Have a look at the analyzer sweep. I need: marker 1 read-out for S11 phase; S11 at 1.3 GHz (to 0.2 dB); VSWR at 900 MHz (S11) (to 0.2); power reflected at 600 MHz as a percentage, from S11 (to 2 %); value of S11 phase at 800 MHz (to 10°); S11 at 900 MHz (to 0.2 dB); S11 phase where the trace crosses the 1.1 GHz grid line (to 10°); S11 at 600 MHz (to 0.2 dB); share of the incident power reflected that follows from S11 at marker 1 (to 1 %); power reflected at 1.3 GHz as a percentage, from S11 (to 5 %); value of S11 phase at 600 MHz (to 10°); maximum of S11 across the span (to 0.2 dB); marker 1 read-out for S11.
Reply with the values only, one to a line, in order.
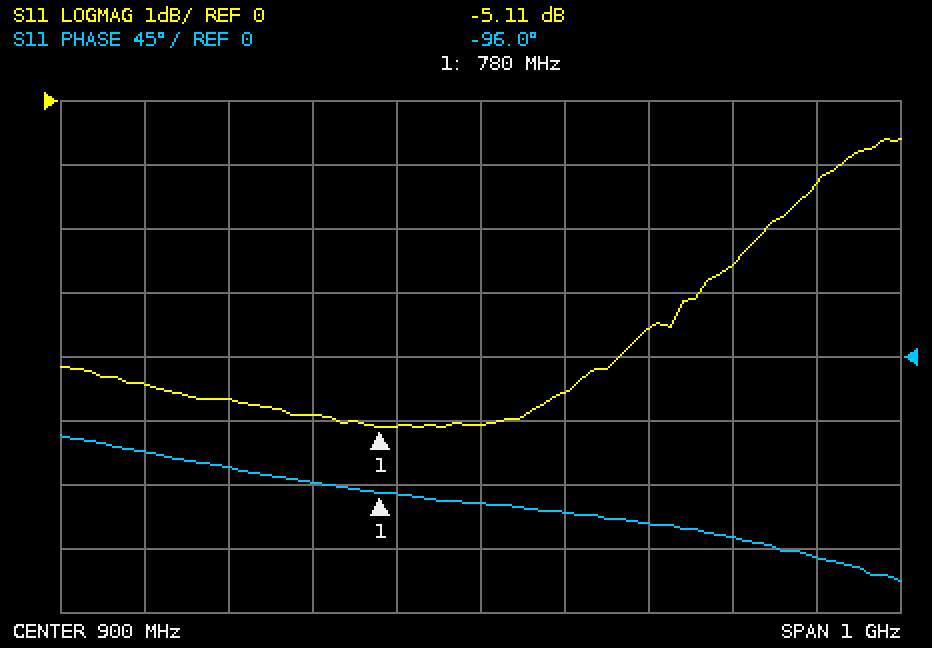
-96.0°
-1.2 dB
3.6
34 %
-100°
-5.0 dB
-120°
-4.6 dB
31 %
75 %
-80°
-0.6 dB
-5.11 dB
